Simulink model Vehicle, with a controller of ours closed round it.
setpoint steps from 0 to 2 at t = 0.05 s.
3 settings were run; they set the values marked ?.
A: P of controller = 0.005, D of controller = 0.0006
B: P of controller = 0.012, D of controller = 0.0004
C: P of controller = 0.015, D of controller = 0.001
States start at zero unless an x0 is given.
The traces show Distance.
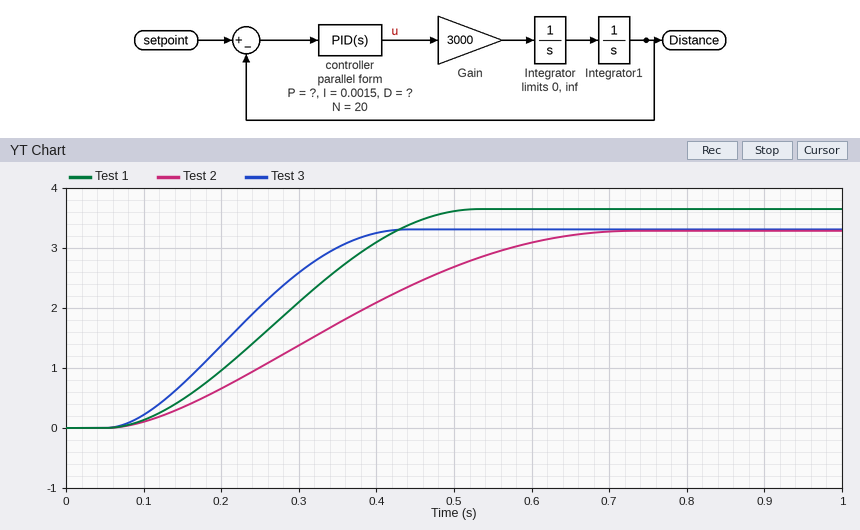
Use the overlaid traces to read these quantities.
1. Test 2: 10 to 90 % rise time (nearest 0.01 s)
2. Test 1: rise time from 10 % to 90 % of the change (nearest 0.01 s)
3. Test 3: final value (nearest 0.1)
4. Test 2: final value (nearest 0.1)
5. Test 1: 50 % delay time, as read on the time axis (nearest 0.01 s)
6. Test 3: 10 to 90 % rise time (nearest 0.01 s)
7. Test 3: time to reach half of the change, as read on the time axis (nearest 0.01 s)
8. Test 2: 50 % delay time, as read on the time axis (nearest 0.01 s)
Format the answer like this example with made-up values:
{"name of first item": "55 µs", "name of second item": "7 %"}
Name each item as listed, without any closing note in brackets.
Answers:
{"Test 2: 10 to 90 % rise time": "0.41 s", "Test 1: rise time from 10 % to 90 % of the change": "0.29 s", "Test 3: final value": "3.3", "Test 2: final value": "3.3", "Test 1: 50 % delay time, as read on the time axis": "0.28 s", "Test 3: 10 to 90 % rise time": "0.23 s", "Test 3: time to reach half of the change, as read on the time axis": "0.22 s", "Test 2: 50 % delay time, as read on the time axis": "0.34 s"}
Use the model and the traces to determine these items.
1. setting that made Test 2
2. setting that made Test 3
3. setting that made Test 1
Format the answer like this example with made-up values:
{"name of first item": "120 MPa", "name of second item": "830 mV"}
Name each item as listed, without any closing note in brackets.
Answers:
{"setting that made Test 2": "A", "setting that made Test 3": "C", "setting that made Test 1": "B"}
